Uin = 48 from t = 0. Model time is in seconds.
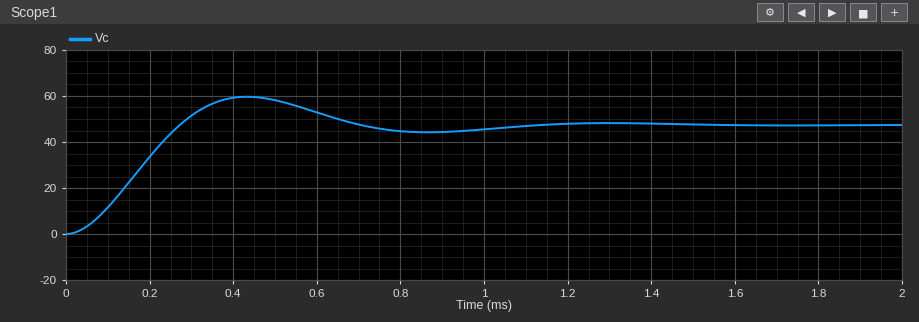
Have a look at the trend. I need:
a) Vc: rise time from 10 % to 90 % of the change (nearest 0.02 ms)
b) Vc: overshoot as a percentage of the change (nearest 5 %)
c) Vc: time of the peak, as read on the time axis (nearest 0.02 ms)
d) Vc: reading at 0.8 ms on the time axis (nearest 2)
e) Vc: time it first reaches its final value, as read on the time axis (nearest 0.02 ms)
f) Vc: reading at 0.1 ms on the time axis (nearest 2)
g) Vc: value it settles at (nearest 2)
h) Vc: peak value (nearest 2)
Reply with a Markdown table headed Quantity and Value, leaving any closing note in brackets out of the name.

| Quantity | Value |
|---|---|
| Vc: rise time from 10 % to 90 % of the change | 0.18 ms |
| Vc: overshoot as a percentage of the change | 25 % |
| Vc: time of the peak, as read on the time axis | 0.44 ms |
| Vc: reading at 0.8 ms on the time axis | 44 |
| Vc: time it first reaches its final value, as read on the time axis | 0.28 ms |
| Vc: reading at 0.1 ms on the time axis | 12 |
| Vc: value it settles at | 48 |
| Vc: peak value | 60 |
